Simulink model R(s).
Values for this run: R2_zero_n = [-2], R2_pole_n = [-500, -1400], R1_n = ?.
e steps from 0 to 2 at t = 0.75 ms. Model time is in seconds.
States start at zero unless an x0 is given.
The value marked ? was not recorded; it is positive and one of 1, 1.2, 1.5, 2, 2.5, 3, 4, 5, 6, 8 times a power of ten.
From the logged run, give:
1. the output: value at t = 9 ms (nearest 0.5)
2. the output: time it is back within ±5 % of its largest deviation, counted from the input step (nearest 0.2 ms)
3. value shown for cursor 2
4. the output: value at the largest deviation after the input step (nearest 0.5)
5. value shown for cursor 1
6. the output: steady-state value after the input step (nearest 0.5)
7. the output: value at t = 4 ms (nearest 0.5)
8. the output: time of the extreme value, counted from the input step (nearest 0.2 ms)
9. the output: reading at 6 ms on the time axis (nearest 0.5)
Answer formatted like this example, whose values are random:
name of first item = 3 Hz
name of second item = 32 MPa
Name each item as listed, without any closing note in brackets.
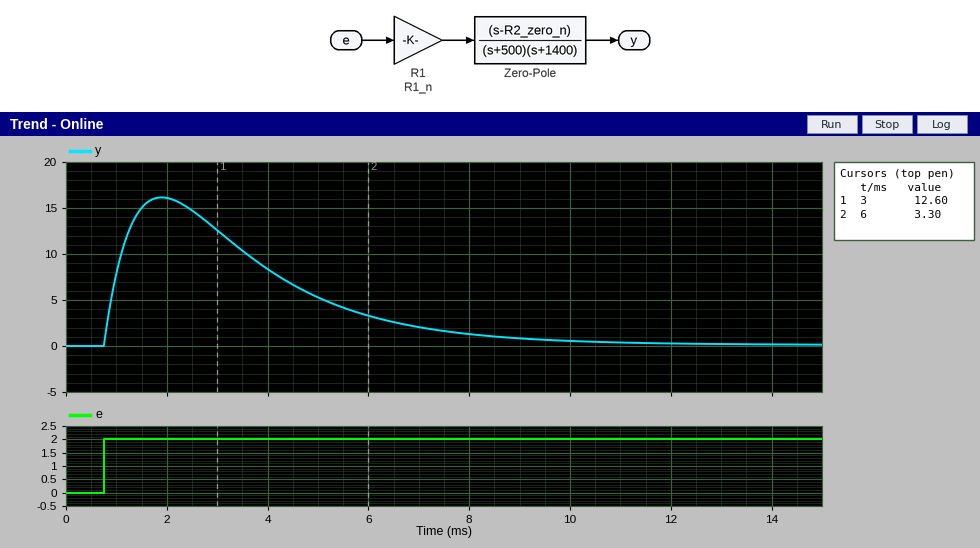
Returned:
the output: value at t = 9 ms = 1.0
the output: time it is back within ±5 % of its largest deviation, counted from the input step = 8.0 ms
value shown for cursor 2 = 3.30
the output: value at the largest deviation after the input step = 16.0
value shown for cursor 1 = 12.60
the output: steady-state value after the input step = 0.0
the output: value at t = 4 ms = 8.5
the output: time of the extreme value, counted from the input step = 1.2 ms
the output: reading at 6 ms on the time axis = 3.5
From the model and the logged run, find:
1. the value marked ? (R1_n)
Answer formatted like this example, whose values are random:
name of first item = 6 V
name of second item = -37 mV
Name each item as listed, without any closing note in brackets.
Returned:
the value marked ? = 20000
